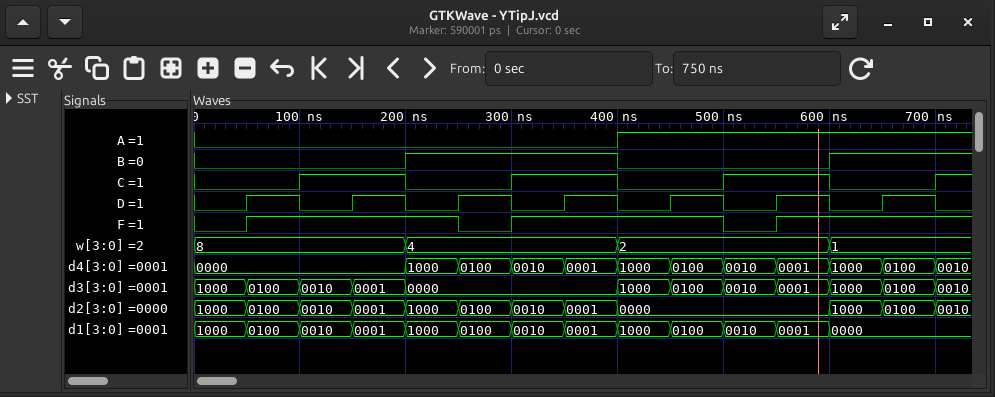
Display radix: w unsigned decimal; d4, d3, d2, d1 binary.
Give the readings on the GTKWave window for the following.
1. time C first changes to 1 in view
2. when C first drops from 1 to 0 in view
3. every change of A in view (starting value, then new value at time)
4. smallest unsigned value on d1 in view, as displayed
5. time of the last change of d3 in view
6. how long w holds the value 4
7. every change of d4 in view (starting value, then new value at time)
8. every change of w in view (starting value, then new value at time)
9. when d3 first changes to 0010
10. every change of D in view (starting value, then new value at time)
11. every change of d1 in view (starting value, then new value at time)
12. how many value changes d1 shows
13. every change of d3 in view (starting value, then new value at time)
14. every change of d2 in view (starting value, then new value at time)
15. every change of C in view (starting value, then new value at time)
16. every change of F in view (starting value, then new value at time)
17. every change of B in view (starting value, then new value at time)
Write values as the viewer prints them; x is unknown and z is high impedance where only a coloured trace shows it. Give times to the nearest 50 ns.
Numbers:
100 ns
200 ns
0, 1 at 400 ns
0000
700 ns
200 ns
0000, 1000 at 200 ns, 0100 at 250 ns, 0010 at 300 ns, 0001 at 350 ns, 1000 at 400 ns, 0100 at 450 ns, 0010 at 500 ns, 0001 at 550 ns, 1000 at 600 ns, 0100 at 650 ns, 0010 at 700 ns
8, 4 at 200 ns, 2 at 400 ns, 1 at 600 ns
100 ns
0, 1 at 50 ns, 0 at 100 ns, 1 at 150 ns, 0 at 200 ns, 1 at 250 ns, 0 at 300 ns, 1 at 350 ns, 0 at 400 ns, 1 at 450 ns, 0 at 500 ns, 1 at 550 ns, 0 at 600 ns, 1 at 650 ns, 0 at 700 ns
1000, 0100 at 50 ns, 0010 at 100 ns, 0001 at 150 ns, 1000 at 200 ns, 0100 at 250 ns, 0010 at 300 ns, 0001 at 350 ns, 1000 at 400 ns, 0100 at 450 ns, 0010 at 500 ns, 0001 at 550 ns, 0000 at 600 ns
12
1000, 0100 at 50 ns, 0010 at 100 ns, 0001 at 150 ns, 0000 at 200 ns, 1000 at 400 ns, 0100 at 450 ns, 0010 at 500 ns, 0001 at 550 ns, 1000 at 600 ns, 0100 at 650 ns, 0010 at 700 ns
1000, 0100 at 50 ns, 0010 at 100 ns, 0001 at 150 ns, 1000 at 200 ns, 0100 at 250 ns, 0010 at 300 ns, 0001 at 350 ns, 0000 at 400 ns, 1000 at 600 ns, 0100 at 650 ns, 0010 at 700 ns
0, 1 at 100 ns, 0 at 200 ns, 1 at 300 ns, 0 at 400 ns, 1 at 500 ns, 0 at 600 ns, 1 at 700 ns
0, 1 at 50 ns, 0 at 250 ns, 1 at 300 ns, 0 at 500 ns, 1 at 550 ns
0, 1 at 200 ns, 0 at 400 ns, 1 at 600 ns
